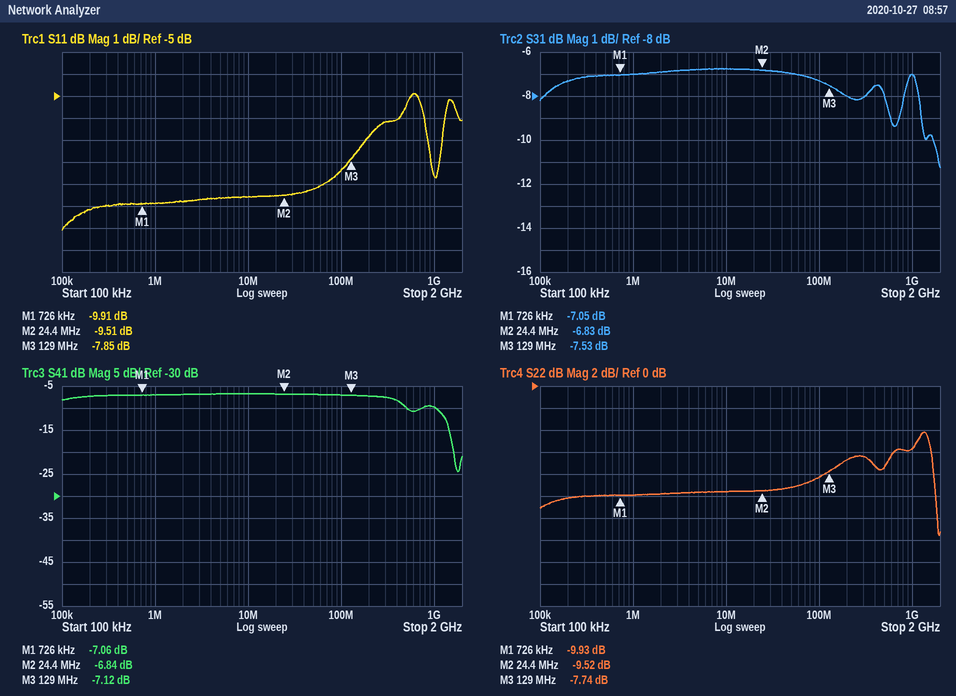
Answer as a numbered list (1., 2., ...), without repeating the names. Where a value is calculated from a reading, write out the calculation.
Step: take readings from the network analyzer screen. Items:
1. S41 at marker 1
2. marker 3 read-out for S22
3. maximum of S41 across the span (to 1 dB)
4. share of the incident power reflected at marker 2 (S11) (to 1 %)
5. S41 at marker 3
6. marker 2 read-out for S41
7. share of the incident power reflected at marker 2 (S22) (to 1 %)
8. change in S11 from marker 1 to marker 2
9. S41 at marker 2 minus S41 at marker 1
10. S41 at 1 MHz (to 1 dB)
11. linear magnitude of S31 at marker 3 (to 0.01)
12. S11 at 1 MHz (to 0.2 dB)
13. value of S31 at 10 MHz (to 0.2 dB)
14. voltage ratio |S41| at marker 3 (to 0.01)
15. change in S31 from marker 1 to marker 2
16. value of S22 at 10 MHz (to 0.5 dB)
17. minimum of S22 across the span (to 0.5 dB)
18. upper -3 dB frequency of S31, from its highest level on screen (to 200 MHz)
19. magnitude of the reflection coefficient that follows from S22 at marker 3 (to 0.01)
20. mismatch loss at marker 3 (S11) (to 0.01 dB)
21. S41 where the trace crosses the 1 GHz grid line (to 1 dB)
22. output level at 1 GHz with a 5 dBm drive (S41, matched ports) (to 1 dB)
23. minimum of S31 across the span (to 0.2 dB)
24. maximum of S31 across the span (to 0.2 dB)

1. -7.06 dB
2. -7.74 dB
3. -7 dB
4. 10^(-9.51/10) ≈ 11 %
5. -7.12 dB
6. -6.84 dB
7. 10^(-9.52/10) ≈ 11 %
8. -9.51 − (-9.91) = 0.40 dB
9. -6.84 − (-7.06) = 0.22 dB
10. -7 dB
11. 10^(-7.53/20) ≈ 0.42
12. -9.8 dB
13. -6.8 dB
14. 10^(-7.12/20) ≈ 0.44
15. -6.83 − (-7.05) = 0.22 dB
16. -9.5 dB
17. -13.5 dB
18. 1.4 GHz
19. 10^(-7.74/20) ≈ 0.41
20. −10 log10(1 − 10^(-7.85/10)) ≈ 0.78 dB
21. -10 dB
22. 5 dBm + (-10 dB) = -5 dBm
23. -11.2 dB
24. -6.8 dB
